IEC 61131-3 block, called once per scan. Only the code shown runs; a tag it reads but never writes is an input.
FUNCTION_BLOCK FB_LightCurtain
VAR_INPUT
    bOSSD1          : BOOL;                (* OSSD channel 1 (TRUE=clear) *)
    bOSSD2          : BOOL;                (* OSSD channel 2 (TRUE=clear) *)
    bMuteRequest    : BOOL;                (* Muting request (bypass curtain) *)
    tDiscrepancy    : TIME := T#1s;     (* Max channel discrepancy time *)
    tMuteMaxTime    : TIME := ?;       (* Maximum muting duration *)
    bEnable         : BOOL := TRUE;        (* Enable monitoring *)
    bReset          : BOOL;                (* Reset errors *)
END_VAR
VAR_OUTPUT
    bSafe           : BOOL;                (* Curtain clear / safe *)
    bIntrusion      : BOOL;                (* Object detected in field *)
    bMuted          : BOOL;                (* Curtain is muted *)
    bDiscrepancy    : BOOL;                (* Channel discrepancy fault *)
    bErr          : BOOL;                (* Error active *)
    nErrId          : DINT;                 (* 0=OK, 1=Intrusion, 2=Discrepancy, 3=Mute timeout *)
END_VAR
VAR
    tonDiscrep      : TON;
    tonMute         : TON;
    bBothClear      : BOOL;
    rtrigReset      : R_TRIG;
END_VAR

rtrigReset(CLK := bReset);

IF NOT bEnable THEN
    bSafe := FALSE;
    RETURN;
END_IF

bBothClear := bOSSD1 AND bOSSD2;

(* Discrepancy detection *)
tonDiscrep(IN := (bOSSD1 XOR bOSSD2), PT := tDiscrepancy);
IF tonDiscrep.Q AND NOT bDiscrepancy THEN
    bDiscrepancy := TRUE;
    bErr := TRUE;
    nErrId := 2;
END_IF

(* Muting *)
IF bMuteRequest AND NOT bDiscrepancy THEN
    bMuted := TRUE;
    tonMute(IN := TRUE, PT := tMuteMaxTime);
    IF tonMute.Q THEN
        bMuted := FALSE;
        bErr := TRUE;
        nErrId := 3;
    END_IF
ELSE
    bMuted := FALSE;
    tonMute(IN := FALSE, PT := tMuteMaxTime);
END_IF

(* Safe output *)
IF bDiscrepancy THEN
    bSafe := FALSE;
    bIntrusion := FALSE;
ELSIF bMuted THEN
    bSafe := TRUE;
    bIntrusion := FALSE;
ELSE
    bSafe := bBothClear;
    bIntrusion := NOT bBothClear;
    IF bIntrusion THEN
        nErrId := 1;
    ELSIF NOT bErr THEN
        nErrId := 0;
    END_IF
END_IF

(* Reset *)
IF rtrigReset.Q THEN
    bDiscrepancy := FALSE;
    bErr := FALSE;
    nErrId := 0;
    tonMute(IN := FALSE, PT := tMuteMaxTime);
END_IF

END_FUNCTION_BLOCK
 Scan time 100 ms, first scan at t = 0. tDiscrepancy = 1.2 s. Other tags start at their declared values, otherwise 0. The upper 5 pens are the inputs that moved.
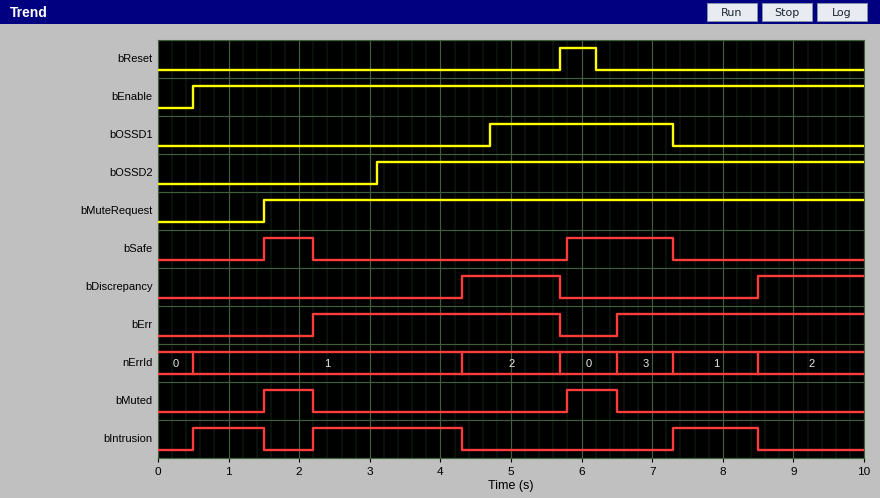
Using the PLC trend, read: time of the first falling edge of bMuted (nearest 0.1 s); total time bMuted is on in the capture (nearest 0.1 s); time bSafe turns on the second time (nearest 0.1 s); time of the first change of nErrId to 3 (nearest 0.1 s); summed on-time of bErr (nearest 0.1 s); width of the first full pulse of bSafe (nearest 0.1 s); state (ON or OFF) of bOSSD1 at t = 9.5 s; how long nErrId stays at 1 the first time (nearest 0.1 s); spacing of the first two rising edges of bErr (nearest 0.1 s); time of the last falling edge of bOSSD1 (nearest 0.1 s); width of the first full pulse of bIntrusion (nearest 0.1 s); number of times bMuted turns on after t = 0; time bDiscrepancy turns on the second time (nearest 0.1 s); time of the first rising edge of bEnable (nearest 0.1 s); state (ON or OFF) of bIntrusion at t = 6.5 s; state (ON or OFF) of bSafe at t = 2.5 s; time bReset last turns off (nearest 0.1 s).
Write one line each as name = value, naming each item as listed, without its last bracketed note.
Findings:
time of the first falling edge of bMuted = 2.2 s
total time bMuted is on in the capture = 1.4 s
time bSafe turns on the second time = 5.8 s
time of the first change of nErrId to 3 = 6.5 s
summed on-time of bErr = 7.0 s
width of the first full pulse of bSafe = 0.7 s
state (ON or OFF) of bOSSD1 at t = 9.5 s = OFF
how long nErrId stays at 1 the first time = 3.8 s
spacing of the first two rising edges of bErr = 4.3 s
time of the last falling edge of bOSSD1 = 7.3 s
width of the first full pulse of bIntrusion = 1.0 s
number of times bMuted turns on after t = 0 = 2
time bDiscrepancy turns on the second time = 8.5 s
time of the first rising edge of bEnable = 0.5 s
state (ON or OFF) of bIntrusion at t = 6.5 s = OFF
state (ON or OFF) of bSafe at t = 2.5 s = OFF
time bReset last turns off = 6.2 s
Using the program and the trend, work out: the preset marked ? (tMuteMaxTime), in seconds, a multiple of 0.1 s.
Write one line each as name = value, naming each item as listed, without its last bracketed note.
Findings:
the preset marked ? (tMuteMaxTime), in seconds, a multiple of 0.1 s = 0.7 s
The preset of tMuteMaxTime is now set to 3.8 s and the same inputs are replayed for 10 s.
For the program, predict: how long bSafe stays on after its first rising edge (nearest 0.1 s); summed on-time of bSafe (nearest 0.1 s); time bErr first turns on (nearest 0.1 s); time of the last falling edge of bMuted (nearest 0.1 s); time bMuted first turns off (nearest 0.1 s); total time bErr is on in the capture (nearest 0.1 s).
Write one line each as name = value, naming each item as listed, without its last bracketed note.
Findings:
how long bSafe stays on after its first rising edge = 2.8 s
summed on-time of bSafe = 5.5 s
time bErr first turns on = 4.3 s
time of the last falling edge of bMuted = 8.5 s
time bMuted first turns off = 4.3 s
total time bErr is on in the capture = 2.9 s
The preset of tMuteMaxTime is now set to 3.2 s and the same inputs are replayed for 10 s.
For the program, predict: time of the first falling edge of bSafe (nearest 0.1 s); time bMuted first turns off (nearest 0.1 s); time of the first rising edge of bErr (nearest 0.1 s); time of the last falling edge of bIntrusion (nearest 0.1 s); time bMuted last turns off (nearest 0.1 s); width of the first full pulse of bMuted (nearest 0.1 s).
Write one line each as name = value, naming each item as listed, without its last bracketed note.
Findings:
time of the first falling edge of bSafe = 4.3 s
time bMuted first turns off = 4.3 s
time of the first rising edge of bErr = 4.3 s
time of the last falling edge of bIntrusion = 1.5 s
time bMuted last turns off = 8.5 s
width of the first full pulse of bMuted = 2.8 s
